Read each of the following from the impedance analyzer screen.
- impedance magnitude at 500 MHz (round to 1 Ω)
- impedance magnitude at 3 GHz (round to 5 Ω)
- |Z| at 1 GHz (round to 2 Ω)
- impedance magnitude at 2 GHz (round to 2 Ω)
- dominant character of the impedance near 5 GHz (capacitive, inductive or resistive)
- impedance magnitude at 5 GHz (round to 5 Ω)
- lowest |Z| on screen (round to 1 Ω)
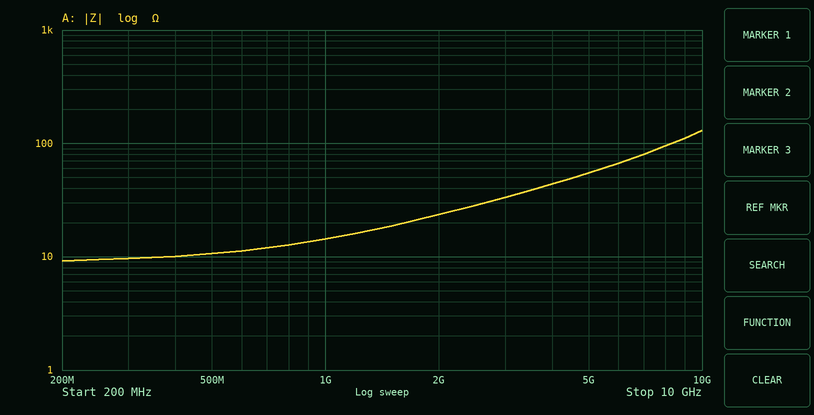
11 Ω
35 Ω
14 Ω
24 Ω
inductive
55 Ω
9 Ω
